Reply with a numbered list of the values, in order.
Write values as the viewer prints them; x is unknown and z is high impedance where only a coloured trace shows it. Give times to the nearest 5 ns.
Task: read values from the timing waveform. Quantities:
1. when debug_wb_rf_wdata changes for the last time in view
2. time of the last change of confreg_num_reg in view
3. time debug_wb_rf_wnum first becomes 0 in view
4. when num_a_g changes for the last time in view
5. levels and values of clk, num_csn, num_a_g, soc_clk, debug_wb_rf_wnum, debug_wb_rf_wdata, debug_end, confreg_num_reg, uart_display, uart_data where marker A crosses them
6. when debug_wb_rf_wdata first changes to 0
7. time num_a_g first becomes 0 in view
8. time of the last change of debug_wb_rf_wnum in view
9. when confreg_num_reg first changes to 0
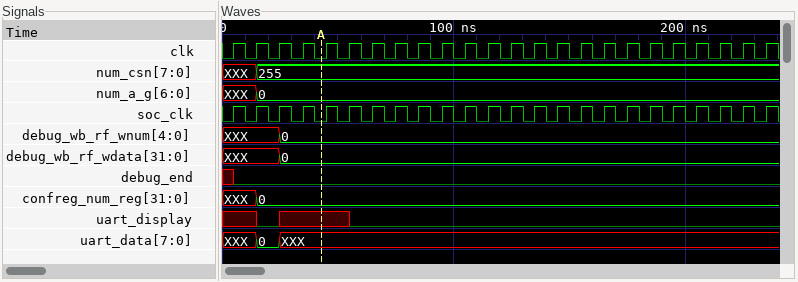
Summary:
1. 25 ns
2. 15 ns
3. 25 ns
4. 15 ns
5. clk=0, num_csn=255, num_a_g=0, soc_clk=0, debug_wb_rf_wnum=0, debug_wb_rf_wdata=0, debug_end=0, confreg_num_reg=0, uart_display=x, uart_data=XXX
6. 25 ns
7. 15 ns
8. 25 ns
9. 15 ns
